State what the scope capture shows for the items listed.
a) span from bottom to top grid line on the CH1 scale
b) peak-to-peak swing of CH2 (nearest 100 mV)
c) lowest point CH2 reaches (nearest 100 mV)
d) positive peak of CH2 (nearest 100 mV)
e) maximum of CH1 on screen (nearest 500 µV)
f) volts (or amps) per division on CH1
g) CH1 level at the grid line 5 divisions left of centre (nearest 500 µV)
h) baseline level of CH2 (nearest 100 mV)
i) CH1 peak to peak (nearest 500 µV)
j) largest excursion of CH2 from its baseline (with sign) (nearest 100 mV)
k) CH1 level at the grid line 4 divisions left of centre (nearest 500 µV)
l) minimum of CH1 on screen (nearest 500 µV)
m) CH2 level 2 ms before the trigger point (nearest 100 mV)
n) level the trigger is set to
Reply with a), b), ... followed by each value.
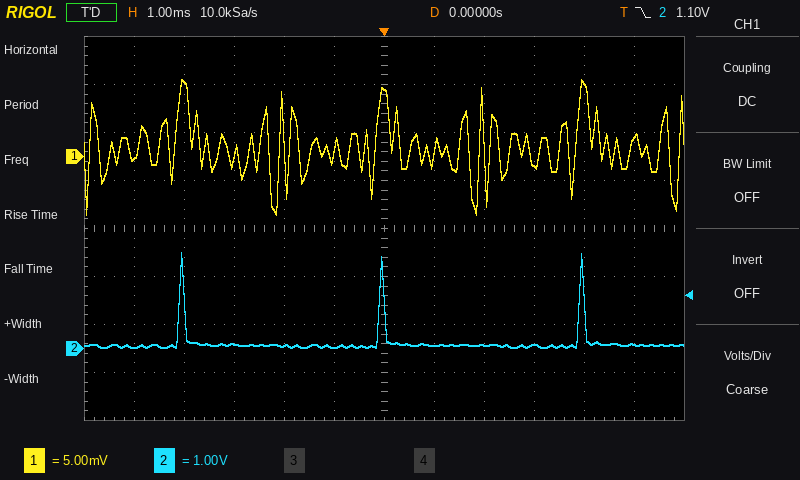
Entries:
a) 40 mV
b) 2.0 V
c) 0.0 V
d) 2.0 V
e) 8.0 mV
f) 5 mV
g) 0.0 mV
h) 100 mV
i) 14.0 mV
j) +1.9 V
k) 7.5 mV
l) -6.0 mV
m) 100 mV
n) 1.10 V
